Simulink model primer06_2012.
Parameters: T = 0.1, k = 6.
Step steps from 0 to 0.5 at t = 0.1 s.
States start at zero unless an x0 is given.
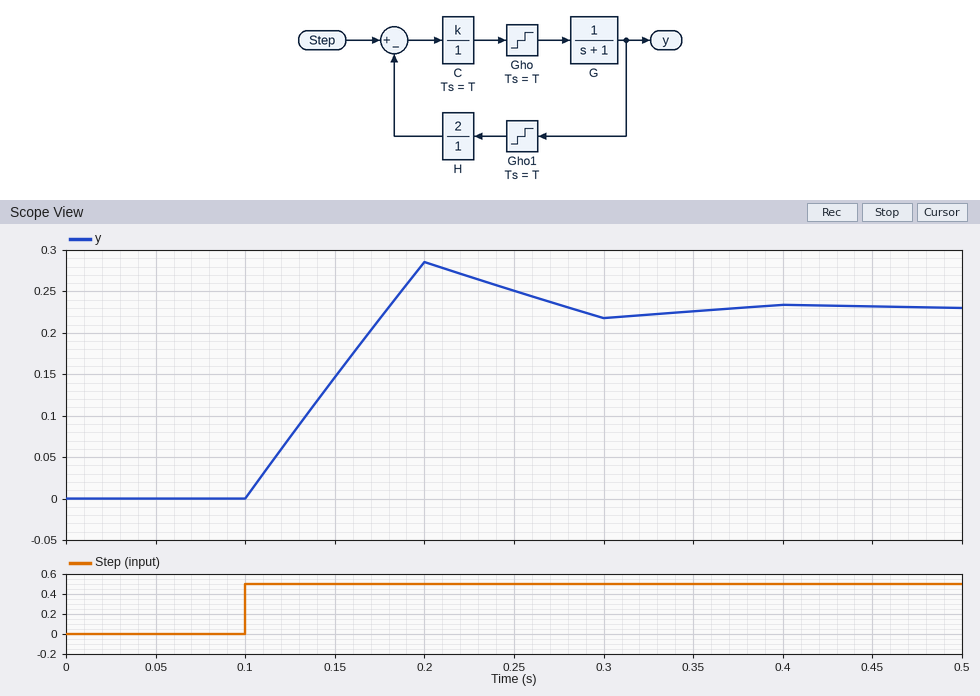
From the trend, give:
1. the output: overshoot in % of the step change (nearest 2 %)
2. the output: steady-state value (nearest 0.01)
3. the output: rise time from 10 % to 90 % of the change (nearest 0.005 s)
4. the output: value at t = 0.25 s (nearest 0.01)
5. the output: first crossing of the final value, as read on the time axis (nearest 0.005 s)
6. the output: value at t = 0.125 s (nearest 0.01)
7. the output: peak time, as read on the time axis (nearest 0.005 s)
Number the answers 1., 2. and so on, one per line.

1. 24 %
2. 0.23
3. 0.065 s
4. 0.25
5. 0.180 s
6. 0.07
7. 0.200 s
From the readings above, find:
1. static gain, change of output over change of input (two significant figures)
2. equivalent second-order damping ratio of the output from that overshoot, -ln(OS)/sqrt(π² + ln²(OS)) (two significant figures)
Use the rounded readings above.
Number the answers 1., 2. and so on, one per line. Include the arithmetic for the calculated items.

1. (0.23 - 0) / (0.5 - 0) = 0.46
2. ln(0.24) = -1.427; 1.427 / sqrt(9.870 + 2.037) = 0.41
